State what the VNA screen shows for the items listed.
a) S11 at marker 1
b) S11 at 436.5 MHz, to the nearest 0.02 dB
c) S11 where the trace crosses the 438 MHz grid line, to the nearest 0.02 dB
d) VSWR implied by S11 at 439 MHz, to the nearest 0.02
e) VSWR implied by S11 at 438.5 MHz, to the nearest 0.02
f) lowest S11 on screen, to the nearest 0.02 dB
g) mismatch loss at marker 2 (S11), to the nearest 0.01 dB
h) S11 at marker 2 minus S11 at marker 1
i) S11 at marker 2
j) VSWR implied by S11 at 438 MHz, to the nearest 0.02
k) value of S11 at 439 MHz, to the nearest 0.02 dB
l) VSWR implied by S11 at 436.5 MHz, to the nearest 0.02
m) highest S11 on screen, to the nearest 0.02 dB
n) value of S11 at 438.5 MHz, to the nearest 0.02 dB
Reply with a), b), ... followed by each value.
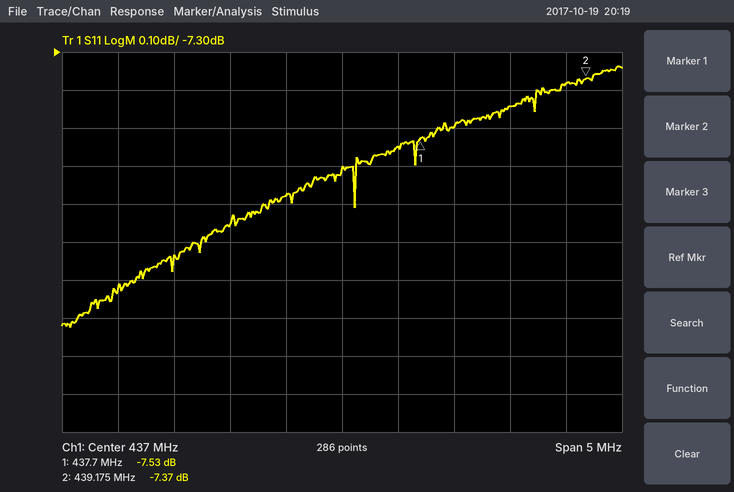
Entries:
a) -7.53 dB
b) -7.68 dB
c) -7.50 dB
d) 2.50
e) 2.48
f) -8.02 dB
g) 0.88 dB
h) 0.16 dB
i) -7.37 dB
j) 2.46
k) -7.38 dB
l) 2.40
m) -7.34 dB
n) -7.44 dB
